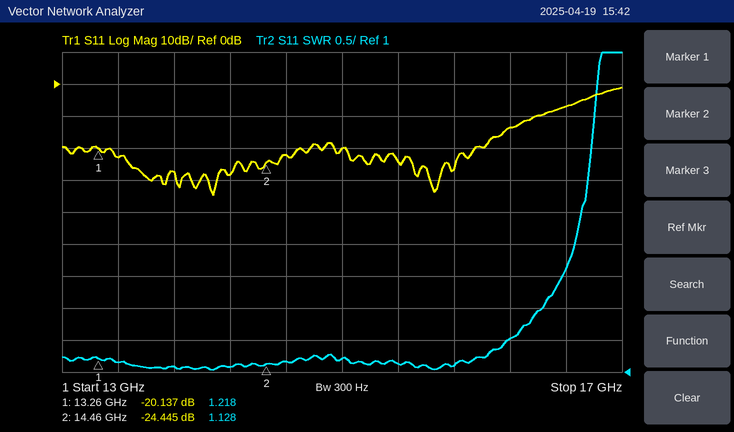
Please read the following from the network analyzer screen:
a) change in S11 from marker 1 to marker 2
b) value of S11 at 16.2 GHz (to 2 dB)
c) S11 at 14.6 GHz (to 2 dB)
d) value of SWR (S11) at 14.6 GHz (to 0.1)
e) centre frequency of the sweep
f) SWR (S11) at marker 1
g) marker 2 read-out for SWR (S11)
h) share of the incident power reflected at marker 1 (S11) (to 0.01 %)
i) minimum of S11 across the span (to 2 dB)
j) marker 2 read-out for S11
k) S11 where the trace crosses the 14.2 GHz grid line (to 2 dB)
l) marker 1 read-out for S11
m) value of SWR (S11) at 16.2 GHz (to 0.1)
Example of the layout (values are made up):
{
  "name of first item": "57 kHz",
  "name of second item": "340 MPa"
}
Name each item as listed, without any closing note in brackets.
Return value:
{
  "change in S11 from marker 1 to marker 2": "-4.308 dB",
  "value of S11 at 16.2 GHz": "-14 dB",
  "S11 at 14.6 GHz": "-22 dB",
  "value of SWR (S11) at 14.6 GHz": "1.2",
  "centre frequency of the sweep": "15 GHz",
  "SWR (S11) at marker 1": "1.218",
  "marker 2 read-out for SWR": "1.128",
  "share of the incident power reflected at marker 1 (S11)": "0.97 %",
  "minimum of S11 across the span": "-34 dB",
  "marker 2 read-out for S11": "-24.445 dB",
  "S11 where the trace crosses the 14.2 GHz grid line": "-28 dB",
  "marker 1 read-out for S11": "-20.137 dB",
  "value of SWR (S11) at 16.2 GHz": "1.5"
}
